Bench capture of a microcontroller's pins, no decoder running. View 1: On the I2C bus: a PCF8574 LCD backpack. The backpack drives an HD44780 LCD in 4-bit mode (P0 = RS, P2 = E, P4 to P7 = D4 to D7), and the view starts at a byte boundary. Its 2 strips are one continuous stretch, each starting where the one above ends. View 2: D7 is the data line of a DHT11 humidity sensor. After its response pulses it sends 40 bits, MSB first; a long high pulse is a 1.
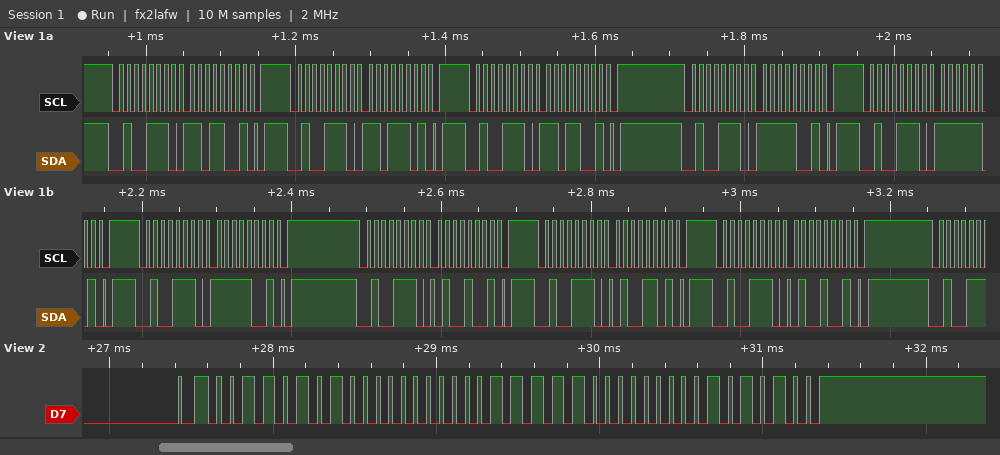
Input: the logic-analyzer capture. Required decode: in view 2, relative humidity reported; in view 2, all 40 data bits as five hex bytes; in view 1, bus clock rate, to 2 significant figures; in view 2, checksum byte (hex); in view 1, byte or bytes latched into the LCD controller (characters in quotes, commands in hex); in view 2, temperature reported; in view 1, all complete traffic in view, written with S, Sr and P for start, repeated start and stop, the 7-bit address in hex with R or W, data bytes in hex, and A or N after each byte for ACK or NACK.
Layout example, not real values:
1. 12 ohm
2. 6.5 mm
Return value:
1. 53 %
2. 35 00 1F 00 54
3. 100 kHz
4. 0x54
5. data 0xDF
6. 31.0 °C
7. S 27W A D9 A P S 27W A DD A P S 27W A D9 A P S 27W A F9 A P S 27W A FD A P S 27W A F9 A P S 27W A 49 A P S 27W A 4D A P S 27W A 49 A P
